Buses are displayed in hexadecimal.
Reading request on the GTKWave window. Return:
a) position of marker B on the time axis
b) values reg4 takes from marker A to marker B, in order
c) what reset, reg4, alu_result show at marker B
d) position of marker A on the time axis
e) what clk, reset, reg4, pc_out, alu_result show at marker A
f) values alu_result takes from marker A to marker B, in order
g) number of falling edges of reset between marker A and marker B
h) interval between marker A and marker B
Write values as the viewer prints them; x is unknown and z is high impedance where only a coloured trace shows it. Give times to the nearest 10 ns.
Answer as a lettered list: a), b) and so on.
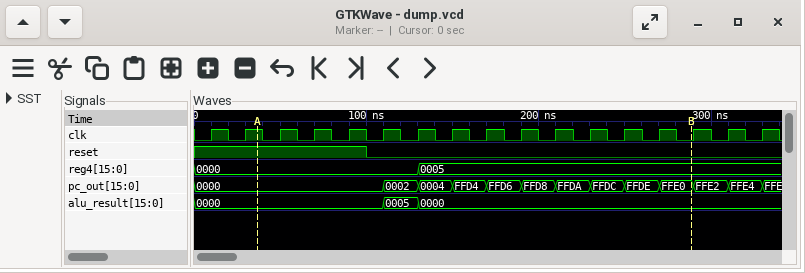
a) 290 ns
b) 0000, 0005
c) reset=0, reg4=0005, alu_result=0000
d) 40 ns
e) clk=1, reset=1, reg4=0000, pc_out=0000, alu_result=0000
f) 0000, 0005, 0000
g) 1
h) 250 ns
